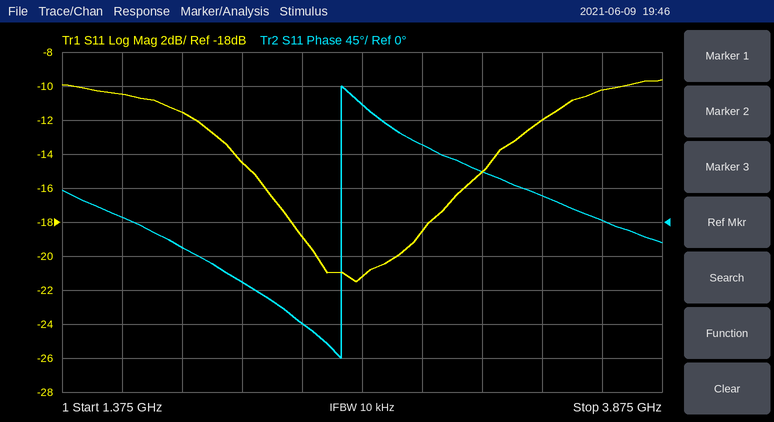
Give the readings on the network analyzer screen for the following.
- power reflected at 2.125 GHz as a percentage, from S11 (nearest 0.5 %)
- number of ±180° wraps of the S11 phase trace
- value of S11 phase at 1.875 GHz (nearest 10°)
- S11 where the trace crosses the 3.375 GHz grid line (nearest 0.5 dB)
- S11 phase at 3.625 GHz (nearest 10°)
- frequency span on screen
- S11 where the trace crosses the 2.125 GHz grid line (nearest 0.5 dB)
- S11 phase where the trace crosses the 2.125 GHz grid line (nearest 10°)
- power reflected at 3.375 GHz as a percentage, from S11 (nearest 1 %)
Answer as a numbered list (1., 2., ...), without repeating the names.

1. 3.5 %
2. 1
3. -30°
4. -12.0 dB
5. 0°
6. 2.5 GHz
7. -14.5 dB
8. -80°
9. 6 %
